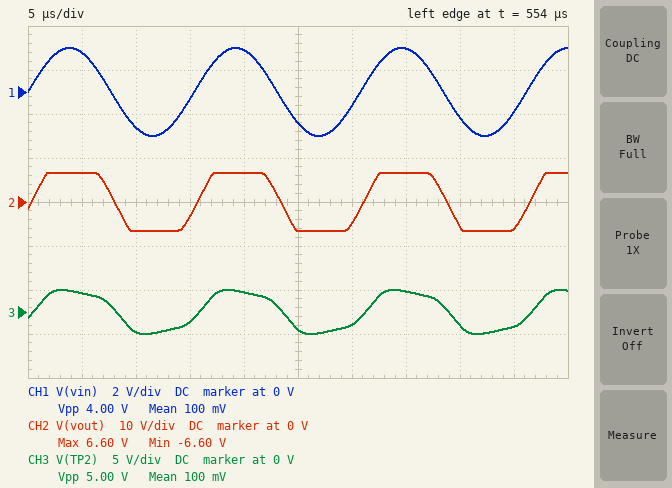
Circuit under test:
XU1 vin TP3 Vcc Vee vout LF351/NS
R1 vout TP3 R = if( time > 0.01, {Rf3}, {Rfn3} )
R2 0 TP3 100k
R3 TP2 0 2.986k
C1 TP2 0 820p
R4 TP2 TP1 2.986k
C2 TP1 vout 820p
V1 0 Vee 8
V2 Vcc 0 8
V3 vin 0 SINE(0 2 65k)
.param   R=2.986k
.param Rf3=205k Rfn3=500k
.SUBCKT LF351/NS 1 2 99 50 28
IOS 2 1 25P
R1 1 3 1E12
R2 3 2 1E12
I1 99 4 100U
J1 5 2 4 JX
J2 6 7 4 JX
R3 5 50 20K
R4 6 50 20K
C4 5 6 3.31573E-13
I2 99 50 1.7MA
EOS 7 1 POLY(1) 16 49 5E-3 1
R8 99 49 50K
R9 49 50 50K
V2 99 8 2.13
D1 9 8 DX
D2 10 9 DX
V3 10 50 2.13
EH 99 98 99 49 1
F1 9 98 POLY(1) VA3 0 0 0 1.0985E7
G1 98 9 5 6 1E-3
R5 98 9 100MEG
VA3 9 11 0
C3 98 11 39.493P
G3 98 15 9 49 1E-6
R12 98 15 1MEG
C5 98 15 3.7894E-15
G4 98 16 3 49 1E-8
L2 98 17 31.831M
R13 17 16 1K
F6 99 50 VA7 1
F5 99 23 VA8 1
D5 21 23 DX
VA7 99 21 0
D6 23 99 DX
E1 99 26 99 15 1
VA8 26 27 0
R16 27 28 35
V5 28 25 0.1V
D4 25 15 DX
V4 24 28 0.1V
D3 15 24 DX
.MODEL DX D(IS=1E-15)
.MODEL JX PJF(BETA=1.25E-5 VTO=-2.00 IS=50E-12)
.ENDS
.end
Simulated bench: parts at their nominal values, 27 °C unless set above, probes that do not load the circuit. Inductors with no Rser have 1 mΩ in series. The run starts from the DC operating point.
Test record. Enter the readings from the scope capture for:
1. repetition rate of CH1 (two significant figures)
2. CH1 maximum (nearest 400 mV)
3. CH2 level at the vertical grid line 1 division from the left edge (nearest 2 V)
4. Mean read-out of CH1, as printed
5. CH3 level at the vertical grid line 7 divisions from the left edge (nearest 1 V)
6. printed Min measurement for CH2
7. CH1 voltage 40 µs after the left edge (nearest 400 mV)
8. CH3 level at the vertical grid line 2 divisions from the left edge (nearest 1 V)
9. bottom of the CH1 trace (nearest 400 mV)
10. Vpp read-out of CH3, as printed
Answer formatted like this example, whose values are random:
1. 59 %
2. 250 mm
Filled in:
1. 65 kHz
2. 2.0 V
3. 6 V
4. 100 mV
5. 2 V
6. -6.60 V
7. -1.2 V
8. -2 V
9. -2.0 V
10. 5.00 V
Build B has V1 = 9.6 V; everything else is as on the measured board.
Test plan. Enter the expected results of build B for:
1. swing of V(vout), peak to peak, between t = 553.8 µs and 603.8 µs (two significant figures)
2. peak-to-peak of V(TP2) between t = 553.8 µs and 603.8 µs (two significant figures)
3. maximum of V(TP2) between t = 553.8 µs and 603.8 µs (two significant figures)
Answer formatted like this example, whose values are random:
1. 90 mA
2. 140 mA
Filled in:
1. 15 V
2. 5.5 V
3. 2.7 V
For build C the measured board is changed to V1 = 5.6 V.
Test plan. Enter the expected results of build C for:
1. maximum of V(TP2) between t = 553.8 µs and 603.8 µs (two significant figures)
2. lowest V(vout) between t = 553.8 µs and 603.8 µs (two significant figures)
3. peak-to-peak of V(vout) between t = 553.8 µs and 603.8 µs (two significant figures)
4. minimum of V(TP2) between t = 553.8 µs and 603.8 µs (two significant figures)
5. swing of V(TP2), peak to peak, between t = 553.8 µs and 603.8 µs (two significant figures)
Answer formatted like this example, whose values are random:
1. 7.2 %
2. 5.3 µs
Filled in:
1. 2.2 V
2. -4.2 V
3. 11 V
4. -2.0 V
5. 4.2 V
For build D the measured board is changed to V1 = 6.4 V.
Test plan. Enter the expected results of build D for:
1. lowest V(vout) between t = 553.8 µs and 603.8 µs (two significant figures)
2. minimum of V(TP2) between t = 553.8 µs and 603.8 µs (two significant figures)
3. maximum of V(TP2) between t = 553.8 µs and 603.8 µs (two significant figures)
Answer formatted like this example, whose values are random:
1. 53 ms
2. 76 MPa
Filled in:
1. -5.0 V
2. -2.2 V
3. 2.3 V
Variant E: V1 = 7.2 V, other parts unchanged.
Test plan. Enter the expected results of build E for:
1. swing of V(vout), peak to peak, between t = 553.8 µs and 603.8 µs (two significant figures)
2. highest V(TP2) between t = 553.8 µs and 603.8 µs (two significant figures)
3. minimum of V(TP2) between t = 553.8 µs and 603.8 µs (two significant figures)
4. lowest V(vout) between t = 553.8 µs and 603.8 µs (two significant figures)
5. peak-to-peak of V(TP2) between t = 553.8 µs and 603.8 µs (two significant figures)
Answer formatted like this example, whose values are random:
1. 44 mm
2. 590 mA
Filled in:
1. 12 V
2. 2.4 V
3. -2.3 V
4. -5.8 V
5. 4.7 V
